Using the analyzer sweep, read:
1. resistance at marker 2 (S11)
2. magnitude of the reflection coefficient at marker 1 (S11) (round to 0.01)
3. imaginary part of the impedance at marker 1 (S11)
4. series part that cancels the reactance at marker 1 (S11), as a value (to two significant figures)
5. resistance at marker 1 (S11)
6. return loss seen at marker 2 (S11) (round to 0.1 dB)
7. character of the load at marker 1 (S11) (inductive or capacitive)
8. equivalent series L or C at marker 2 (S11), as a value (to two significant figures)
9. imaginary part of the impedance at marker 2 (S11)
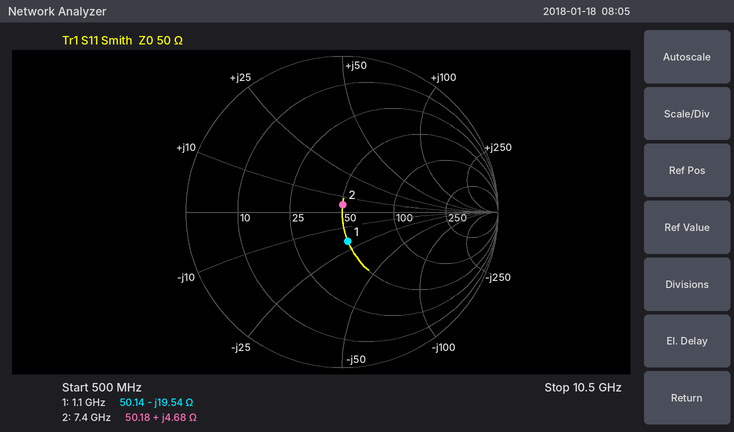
50.18 Ω
0.19
-19.54 Ω
2.8 nH
50.14 Ω
26.6 dB
capacitive
100 pH
+4.68 Ω
